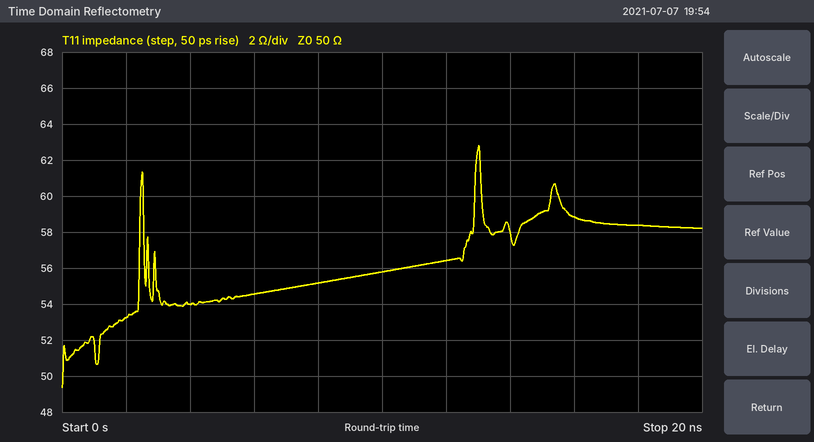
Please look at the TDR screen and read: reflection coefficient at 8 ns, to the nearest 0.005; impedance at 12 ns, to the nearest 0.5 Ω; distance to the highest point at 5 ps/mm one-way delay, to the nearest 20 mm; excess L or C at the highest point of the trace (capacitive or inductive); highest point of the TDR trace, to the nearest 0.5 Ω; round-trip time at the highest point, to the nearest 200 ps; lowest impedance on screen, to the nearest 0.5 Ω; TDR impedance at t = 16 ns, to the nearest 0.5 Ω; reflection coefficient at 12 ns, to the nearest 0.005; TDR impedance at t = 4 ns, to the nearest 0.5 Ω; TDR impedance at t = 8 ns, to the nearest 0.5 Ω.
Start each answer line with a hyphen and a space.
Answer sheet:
- +0.050
- 56.5 Ω
- 1.30 m
- inductive
- 63.0 Ω
- 13.0 ns
- 49.5 Ω
- 59.0 Ω
- +0.060
- 54.0 Ω
- 55.0 Ω
